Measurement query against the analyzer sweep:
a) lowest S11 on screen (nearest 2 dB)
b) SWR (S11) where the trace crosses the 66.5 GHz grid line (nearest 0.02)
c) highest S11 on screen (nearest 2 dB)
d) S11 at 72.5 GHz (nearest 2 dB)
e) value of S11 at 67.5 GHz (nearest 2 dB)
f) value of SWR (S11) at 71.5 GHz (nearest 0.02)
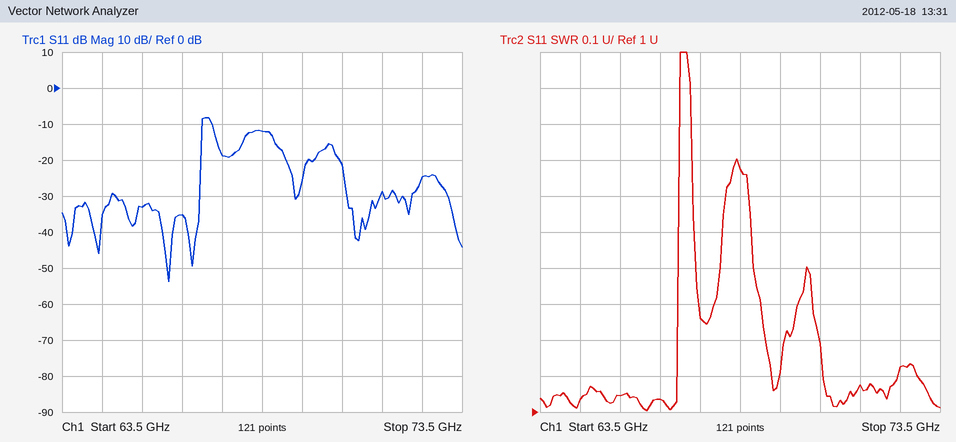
-54 dB
1.04
-8 dB
-24 dB
-18 dB
1.08
